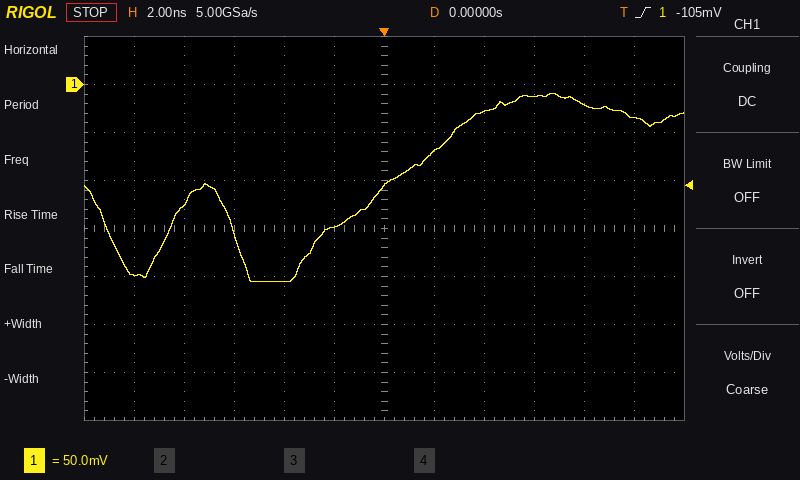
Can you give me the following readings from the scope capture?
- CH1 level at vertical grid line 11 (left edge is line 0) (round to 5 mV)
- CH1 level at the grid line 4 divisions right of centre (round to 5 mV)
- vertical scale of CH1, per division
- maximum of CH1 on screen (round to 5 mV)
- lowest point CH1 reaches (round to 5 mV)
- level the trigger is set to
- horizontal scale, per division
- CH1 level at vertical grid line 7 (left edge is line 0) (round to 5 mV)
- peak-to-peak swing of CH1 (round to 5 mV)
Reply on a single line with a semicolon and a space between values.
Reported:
-35 mV; -20 mV; 50 mV; -10 mV; -205 mV; -105 mV; 2 ns; -70 mV; 195 mV
